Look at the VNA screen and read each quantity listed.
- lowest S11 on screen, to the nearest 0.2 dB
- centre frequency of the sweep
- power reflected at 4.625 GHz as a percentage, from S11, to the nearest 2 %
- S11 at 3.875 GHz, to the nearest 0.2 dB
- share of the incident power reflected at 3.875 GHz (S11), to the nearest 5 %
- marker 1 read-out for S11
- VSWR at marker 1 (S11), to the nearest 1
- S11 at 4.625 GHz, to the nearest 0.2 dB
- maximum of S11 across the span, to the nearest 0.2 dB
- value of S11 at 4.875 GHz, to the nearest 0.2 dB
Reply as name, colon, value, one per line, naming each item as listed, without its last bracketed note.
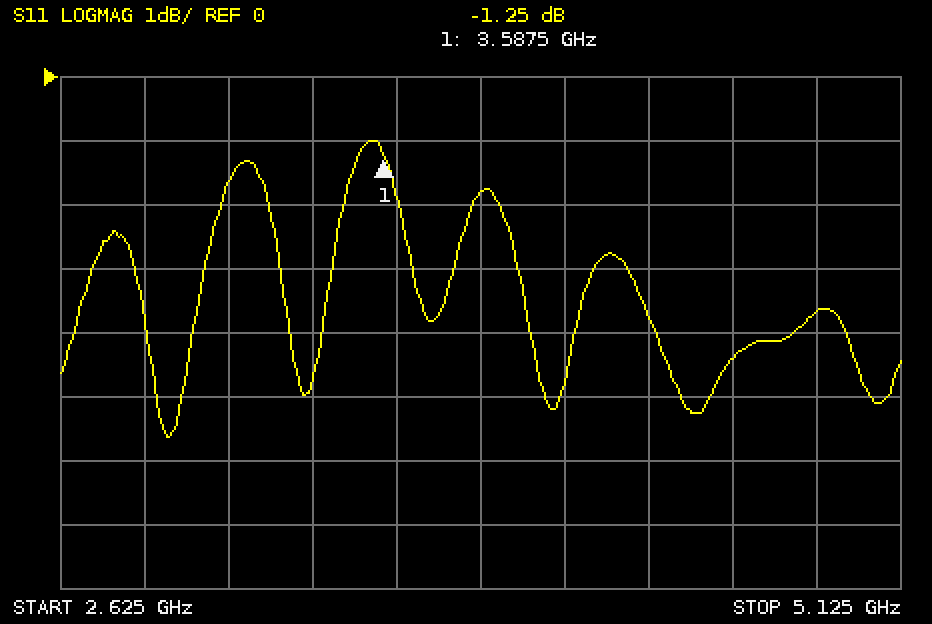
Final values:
lowest S11 on screen, to the nearest 0.2 dB: -5.6 dB
centre frequency of the sweep: 3.875 GHz
power reflected at 4.625 GHz as a percentage, from S11, to the nearest 2 %: 36 %
S11 at 3.875 GHz, to the nearest 0.2 dB: -1.8 dB
share of the incident power reflected at 3.875 GHz (S11), to the nearest 5 %: 65 %
marker 1 read-out for S11: -1.25 dB
VSWR at marker 1 (S11), to the nearest 1: 14
S11 at 4.625 GHz, to the nearest 0.2 dB: -4.4 dB
maximum of S11 across the span, to the nearest 0.2 dB: -1.0 dB
value of S11 at 4.875 GHz, to the nearest 0.2 dB: -3.6 dB
